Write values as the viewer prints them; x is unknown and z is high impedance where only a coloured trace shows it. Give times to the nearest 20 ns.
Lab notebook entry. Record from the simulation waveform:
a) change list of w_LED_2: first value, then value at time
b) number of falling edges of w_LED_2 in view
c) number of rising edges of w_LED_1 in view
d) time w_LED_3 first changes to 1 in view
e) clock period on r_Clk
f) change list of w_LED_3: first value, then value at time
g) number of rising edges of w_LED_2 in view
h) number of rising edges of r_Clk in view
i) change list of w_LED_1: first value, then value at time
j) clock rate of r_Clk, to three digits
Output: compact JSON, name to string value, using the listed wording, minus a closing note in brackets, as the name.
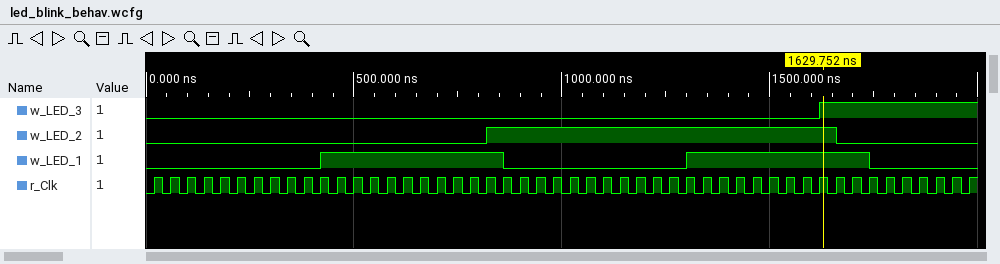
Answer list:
{"change list of w_LED_2: first value, then value at time": "0, 1 at 820 ns, 0 at 1660 ns", "number of falling edges of w_LED_2 in view": "1", "number of rising edges of w_LED_1 in view": "2", "time w_LED_3 first changes to 1 in view": "1620 ns", "clock period on r_Clk": "40 ns", "change list of w_LED_3: first value, then value at time": "0, 1 at 1620 ns", "number of rising edges of w_LED_2 in view": "1", "number of rising edges of r_Clk in view": "50", "change list of w_LED_1: first value, then value at time": "0, 1 at 420 ns, 0 at 860 ns, 1 at 1300 ns, 0 at 1740 ns", "clock rate of r_Clk, to three digits": "25.0 MHz"}
